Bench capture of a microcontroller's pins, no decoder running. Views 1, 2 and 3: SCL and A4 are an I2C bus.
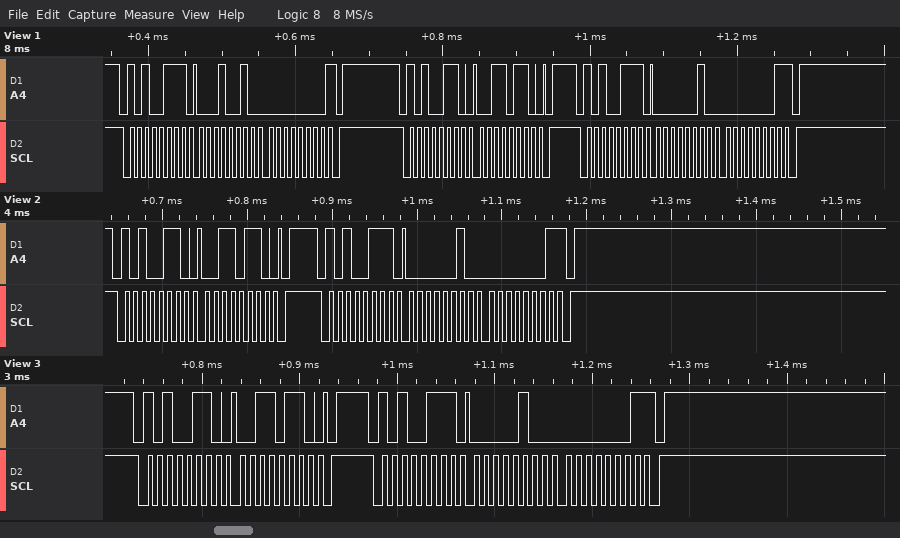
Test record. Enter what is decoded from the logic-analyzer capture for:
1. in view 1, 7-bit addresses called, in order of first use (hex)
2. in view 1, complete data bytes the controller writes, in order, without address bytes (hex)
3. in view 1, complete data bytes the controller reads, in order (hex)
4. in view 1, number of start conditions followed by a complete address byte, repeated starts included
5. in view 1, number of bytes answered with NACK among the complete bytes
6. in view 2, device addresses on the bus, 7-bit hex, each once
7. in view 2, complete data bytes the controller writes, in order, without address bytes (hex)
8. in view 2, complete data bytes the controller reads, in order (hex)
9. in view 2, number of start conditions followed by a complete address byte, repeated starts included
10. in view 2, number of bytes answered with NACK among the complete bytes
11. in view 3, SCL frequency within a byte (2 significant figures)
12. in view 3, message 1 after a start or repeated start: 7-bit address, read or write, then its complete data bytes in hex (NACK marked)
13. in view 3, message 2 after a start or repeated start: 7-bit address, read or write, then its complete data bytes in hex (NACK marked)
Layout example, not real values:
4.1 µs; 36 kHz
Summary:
0x53; 36; 12 00 02 01; 3; 2; 0x53; 36; 02 01; 2; 1; 100 kHz; 0x53 write: 36; 0x53 read: 04 01 NACK
